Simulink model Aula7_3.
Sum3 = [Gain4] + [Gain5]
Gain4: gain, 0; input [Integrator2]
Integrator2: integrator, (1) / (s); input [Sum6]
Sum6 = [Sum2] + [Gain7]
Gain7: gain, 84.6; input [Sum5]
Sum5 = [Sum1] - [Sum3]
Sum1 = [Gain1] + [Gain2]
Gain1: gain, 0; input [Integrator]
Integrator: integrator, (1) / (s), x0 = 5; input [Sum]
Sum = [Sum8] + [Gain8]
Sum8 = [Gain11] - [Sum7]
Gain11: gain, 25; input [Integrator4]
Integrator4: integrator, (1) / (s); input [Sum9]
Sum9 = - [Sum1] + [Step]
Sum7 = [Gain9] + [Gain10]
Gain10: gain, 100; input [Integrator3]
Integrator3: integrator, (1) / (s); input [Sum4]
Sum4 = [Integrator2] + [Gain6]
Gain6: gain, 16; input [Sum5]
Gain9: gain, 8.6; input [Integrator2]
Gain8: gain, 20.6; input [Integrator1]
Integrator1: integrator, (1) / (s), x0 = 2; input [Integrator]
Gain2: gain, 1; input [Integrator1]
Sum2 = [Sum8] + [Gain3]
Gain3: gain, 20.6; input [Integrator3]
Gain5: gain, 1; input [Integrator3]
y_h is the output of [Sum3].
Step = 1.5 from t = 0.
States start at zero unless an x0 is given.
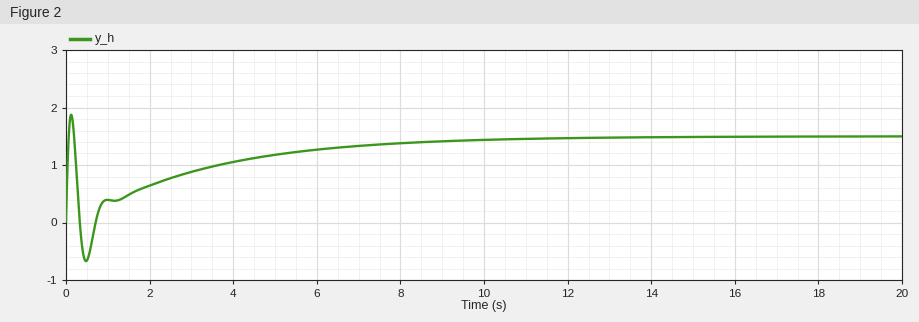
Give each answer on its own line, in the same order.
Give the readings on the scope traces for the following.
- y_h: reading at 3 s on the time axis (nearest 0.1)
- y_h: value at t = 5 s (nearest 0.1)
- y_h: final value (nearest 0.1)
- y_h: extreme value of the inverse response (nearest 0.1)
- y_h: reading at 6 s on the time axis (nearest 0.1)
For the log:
0.9
1.2
1.5
-0.7
1.3
